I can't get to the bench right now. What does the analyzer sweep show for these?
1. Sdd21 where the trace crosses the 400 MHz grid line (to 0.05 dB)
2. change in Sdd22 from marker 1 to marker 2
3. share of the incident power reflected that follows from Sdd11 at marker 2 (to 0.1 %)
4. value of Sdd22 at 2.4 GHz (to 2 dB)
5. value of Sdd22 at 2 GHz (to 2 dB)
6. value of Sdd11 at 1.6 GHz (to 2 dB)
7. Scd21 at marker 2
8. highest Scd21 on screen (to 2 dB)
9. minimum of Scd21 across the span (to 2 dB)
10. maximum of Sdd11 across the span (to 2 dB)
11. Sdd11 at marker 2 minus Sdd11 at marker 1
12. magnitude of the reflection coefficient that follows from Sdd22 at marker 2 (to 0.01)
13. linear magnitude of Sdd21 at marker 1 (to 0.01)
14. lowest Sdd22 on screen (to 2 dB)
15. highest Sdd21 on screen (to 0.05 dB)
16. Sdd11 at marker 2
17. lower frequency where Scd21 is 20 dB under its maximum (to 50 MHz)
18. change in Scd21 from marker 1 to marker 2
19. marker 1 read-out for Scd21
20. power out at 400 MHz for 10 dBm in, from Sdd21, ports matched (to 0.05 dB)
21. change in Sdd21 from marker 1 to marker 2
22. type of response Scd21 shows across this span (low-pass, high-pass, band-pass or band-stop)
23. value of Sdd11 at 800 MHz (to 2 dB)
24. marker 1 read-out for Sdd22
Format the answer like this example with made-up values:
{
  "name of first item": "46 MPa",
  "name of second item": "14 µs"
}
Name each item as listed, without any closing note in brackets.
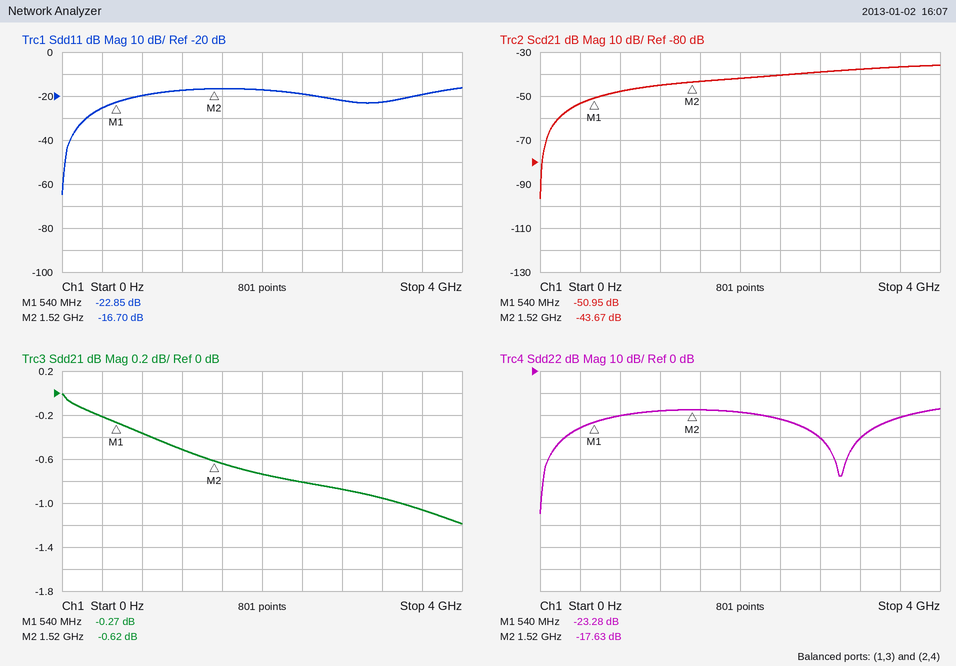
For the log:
{
  "Sdd21 where the trace crosses the 400 MHz grid line": "-0.20 dB",
  "change in Sdd22 from marker 1 to marker 2": "5.65 dB",
  "share of the incident power reflected that follows from Sdd11 at marker 2": "2.1 %",
  "value of Sdd22 at 2.4 GHz": "-22 dB",
  "value of Sdd22 at 2 GHz": "-18 dB",
  "value of Sdd11 at 1.6 GHz": "-16 dB",
  "Scd21 at marker 2": "-43.67 dB",
  "highest Scd21 on screen": "-36 dB",
  "minimum of Scd21 across the span": "-96 dB",
  "maximum of Sdd11 across the span": "-16 dB",
  "Sdd11 at marker 2 minus Sdd11 at marker 1": "6.15 dB",
  "magnitude of the reflection coefficient that follows from Sdd22 at marker 2": "0.13",
  "linear magnitude of Sdd21 at marker 1": "0.97",
  "lowest Sdd22 on screen": "-64 dB",
  "highest Sdd21 on screen": "0.00 dB",
  "Sdd11 at marker 2": "-16.70 dB",
  "lower frequency where Scd21 is 20 dB under its maximum": "300 MHz",
  "change in Scd21 from marker 1 to marker 2": "7.28 dB",
  "marker 1 read-out for Scd21": "-50.95 dB",
  "power out at 400 MHz for 10 dBm in, from Sdd21, ports matched": "9.80 dBm",
  "change in Sdd21 from marker 1 to marker 2": "-0.35 dB",
  "type of response Scd21 shows across this span": "high-pass",
  "value of Sdd11 at 800 MHz": "-20 dB",
  "marker 1 read-out for Sdd22": "-23.28 dB"
}
